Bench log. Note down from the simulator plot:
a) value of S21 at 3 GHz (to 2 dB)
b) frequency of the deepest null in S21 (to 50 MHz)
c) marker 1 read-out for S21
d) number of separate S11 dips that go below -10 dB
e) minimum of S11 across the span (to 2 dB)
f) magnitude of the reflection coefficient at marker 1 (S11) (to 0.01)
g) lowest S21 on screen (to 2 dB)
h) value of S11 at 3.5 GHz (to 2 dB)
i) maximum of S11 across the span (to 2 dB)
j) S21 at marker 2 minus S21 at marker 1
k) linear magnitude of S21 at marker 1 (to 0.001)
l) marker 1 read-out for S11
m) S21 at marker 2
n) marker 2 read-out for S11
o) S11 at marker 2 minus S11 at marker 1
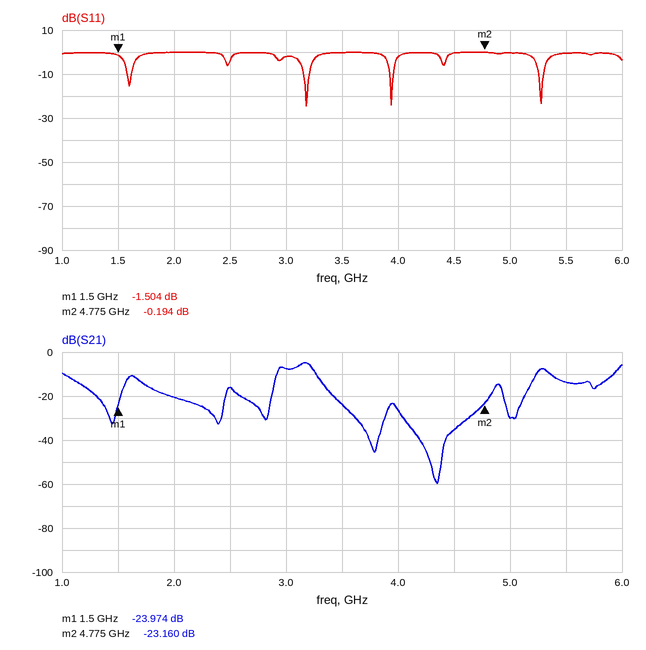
-8 dB
4.35 GHz
-23.974 dB
4
-24 dB
0.84
-60 dB
0 dB
0 dB
0.814 dB
0.063
-1.504 dB
-23.160 dB
-0.194 dB
1.310 dB
